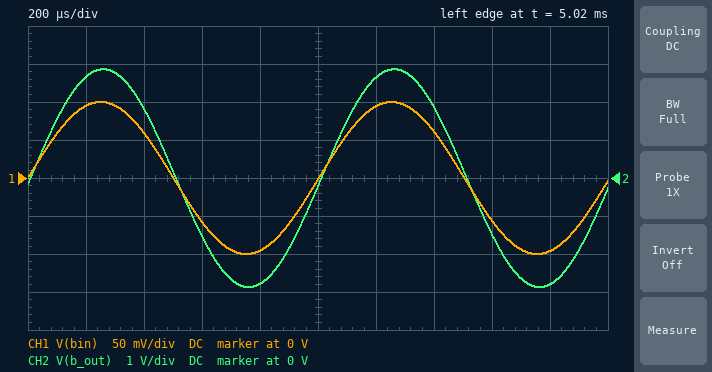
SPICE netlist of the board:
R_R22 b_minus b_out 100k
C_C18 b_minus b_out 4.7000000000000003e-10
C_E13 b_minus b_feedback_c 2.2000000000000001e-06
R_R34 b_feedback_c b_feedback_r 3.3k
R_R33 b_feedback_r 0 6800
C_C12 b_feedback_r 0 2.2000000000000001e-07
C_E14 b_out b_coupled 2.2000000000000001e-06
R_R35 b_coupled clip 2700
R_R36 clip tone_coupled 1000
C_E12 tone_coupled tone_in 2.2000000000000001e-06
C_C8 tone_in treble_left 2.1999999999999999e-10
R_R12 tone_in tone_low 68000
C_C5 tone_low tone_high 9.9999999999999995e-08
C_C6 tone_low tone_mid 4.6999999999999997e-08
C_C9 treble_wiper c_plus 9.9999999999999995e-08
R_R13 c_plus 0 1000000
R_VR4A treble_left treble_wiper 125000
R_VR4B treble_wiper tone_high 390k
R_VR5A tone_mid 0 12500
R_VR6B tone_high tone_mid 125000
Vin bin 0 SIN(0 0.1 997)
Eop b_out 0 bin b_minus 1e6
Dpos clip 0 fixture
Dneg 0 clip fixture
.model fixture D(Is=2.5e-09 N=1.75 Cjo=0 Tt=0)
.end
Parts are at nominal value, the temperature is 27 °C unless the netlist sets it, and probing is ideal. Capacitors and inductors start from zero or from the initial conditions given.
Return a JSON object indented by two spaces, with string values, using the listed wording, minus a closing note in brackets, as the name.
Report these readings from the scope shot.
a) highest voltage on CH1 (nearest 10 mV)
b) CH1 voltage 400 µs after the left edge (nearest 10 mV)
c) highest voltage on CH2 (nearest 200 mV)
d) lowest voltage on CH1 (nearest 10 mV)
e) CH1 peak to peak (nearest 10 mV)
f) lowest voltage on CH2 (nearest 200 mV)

{
  "highest voltage on CH1": "100 mV",
  "CH1 voltage 400 µs after the left edge": "60 mV",
  "highest voltage on CH2": "2.8 V",
  "lowest voltage on CH1": "-100 mV",
  "CH1 peak to peak": "200 mV",
  "lowest voltage on CH2": "-2.8 V"
}
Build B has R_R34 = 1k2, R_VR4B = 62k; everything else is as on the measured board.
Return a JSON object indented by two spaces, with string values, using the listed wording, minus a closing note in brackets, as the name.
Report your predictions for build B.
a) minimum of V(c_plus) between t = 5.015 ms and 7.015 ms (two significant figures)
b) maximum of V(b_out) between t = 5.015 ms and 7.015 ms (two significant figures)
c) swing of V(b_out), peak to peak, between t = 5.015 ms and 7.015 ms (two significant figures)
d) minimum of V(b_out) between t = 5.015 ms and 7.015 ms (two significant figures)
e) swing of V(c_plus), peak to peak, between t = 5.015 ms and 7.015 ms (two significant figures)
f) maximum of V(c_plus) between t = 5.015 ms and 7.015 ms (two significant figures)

{
  "minimum of V(c_plus) between t = 5.015 ms and 7.015 ms": "-240 mV",
  "maximum of V(b_out) between t = 5.015 ms and 7.015 ms": "6.5 V",
  "swing of V(b_out), peak to peak, between t = 5.015 ms and 7.015 ms": "13 V",
  "minimum of V(b_out) between t = 5.015 ms and 7.015 ms": "-6.5 V",
  "swing of V(c_plus), peak to peak, between t = 5.015 ms and 7.015 ms": "480 mV",
  "maximum of V(c_plus) between t = 5.015 ms and 7.015 ms": "240 mV"
}
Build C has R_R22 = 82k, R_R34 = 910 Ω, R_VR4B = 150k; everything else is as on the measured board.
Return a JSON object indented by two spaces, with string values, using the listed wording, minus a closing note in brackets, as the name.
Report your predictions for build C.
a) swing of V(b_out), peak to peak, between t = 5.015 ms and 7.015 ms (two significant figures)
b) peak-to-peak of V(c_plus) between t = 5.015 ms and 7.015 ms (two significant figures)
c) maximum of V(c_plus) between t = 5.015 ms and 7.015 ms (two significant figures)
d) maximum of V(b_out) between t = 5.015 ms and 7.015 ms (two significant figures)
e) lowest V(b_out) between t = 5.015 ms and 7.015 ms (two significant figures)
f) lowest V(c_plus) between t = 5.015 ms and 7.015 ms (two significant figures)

{
  "swing of V(b_out), peak to peak, between t = 5.015 ms and 7.015 ms": "13 V",
  "peak-to-peak of V(c_plus) between t = 5.015 ms and 7.015 ms": "750 mV",
  "maximum of V(c_plus) between t = 5.015 ms and 7.015 ms": "370 mV",
  "maximum of V(b_out) between t = 5.015 ms and 7.015 ms": "6.4 V",
  "lowest V(b_out) between t = 5.015 ms and 7.015 ms": "-6.4 V",
  "lowest V(c_plus) between t = 5.015 ms and 7.015 ms": "-380 mV"
}
